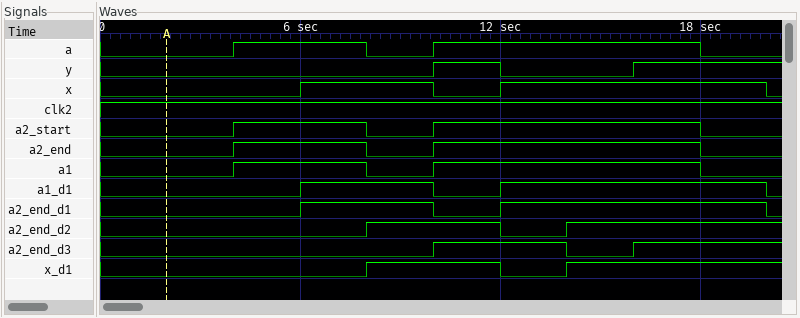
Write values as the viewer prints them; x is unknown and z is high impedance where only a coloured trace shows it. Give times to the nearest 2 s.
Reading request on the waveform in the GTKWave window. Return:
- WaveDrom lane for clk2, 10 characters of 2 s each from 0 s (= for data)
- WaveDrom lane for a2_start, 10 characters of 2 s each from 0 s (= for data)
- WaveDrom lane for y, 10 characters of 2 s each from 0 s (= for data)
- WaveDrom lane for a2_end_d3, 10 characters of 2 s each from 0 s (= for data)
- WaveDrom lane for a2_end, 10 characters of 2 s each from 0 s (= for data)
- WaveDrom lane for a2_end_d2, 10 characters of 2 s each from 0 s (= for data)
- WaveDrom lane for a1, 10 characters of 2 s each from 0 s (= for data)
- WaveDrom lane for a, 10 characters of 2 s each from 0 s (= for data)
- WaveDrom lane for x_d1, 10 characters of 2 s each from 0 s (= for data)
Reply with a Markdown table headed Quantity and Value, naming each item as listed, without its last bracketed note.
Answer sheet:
| Quantity | Value |
|---|---|
| WaveDrom lane for clk2, 10 characters of 2 s each from 0 s | {name: 'clk2', wave: '1.........'} |
| WaveDrom lane for a2_start, 10 characters of 2 s each from 0 s | {name: 'a2_start', wave: '0.1.01...0'} |
| WaveDrom lane for y, 10 characters of 2 s each from 0 s | {name: 'y', wave: '0....10.1.'} |
| WaveDrom lane for a2_end_d3, 10 characters of 2 s each from 0 s | {name: 'a2_end_d3', wave: '0....1.01.'} |
| WaveDrom lane for a2_end, 10 characters of 2 s each from 0 s | {name: 'a2_end', wave: '0.1.01...0'} |
| WaveDrom lane for a2_end_d2, 10 characters of 2 s each from 0 s | {name: 'a2_end_d2', wave: '0...1.01..'} |
| WaveDrom lane for a1, 10 characters of 2 s each from 0 s | {name: 'a1', wave: '0.1.01...0'} |
| WaveDrom lane for a, 10 characters of 2 s each from 0 s | {name: 'a', wave: '0.1.01...0'} |
| WaveDrom lane for x_d1, 10 characters of 2 s each from 0 s | {name: 'x_d1', wave: '0...1.01..'} |
